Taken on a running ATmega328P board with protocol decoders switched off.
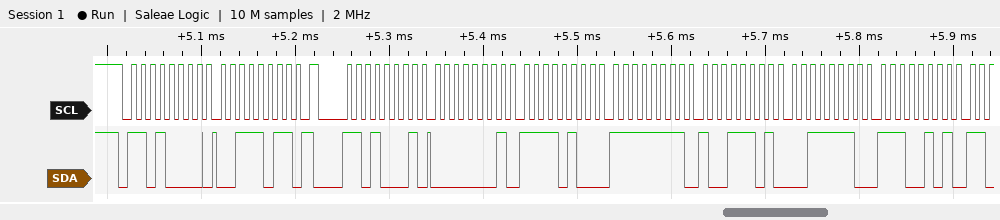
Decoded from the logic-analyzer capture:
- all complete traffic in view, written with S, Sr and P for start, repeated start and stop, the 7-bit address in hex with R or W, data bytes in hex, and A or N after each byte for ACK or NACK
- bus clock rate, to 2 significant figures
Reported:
S 68W A 3B A Sr 68R A 01 A F4 A FF A 9D A 3E A E5 A
100 kHz
